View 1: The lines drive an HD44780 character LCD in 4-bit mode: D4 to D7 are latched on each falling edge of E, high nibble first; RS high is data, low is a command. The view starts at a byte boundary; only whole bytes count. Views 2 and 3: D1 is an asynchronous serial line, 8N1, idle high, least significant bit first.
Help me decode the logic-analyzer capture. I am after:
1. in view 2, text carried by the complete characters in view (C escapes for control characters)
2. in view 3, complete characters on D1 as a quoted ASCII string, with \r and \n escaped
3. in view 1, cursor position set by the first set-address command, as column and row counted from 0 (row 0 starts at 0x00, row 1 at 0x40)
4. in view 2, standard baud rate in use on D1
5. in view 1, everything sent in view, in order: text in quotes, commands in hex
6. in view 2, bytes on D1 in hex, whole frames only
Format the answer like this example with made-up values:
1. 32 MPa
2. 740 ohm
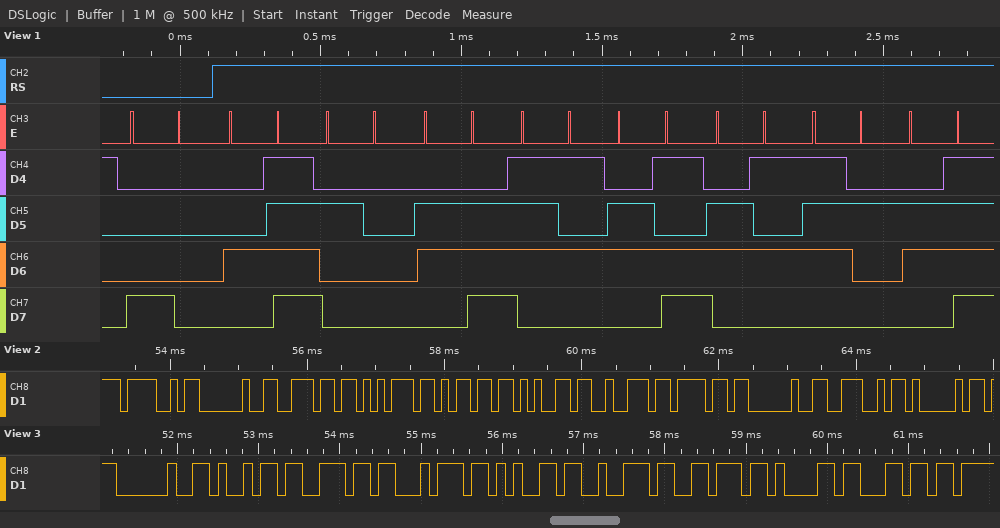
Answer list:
1. "O numero NA"
2. " interval"
3. column 0, row 0
4. 9600 baud
5. 0x80 "O numero"
6. 4F 20 6E 75 6D 65 72 6F 20 4E 41
